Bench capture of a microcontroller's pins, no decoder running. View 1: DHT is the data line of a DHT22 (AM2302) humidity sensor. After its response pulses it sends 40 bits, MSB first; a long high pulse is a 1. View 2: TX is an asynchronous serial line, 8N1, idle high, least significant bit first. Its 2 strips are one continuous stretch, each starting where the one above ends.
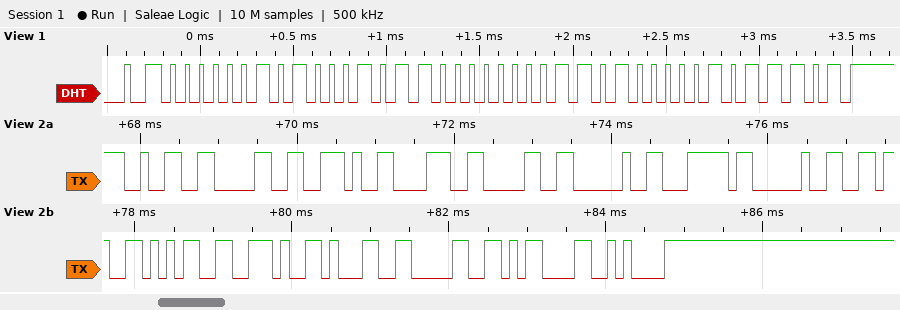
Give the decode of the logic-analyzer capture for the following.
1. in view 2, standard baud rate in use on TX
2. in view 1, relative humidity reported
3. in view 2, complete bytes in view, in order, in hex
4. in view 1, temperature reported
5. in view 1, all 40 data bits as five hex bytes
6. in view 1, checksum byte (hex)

9600 baud
65.1 %
32 30 2E 38 30 20 7C 20 36 35 2E 31 30 0D 0A
20.8 °C
02 8B 00 D0 5D
0x5D
